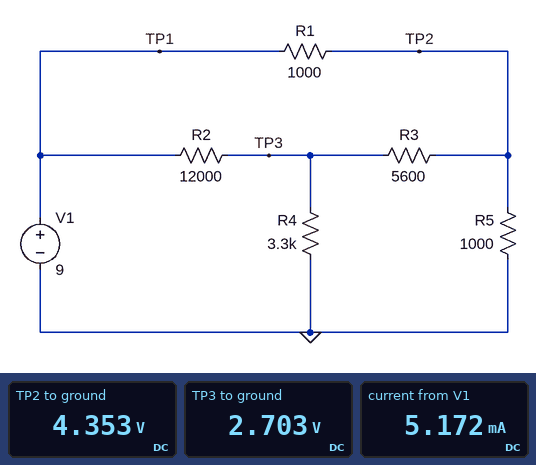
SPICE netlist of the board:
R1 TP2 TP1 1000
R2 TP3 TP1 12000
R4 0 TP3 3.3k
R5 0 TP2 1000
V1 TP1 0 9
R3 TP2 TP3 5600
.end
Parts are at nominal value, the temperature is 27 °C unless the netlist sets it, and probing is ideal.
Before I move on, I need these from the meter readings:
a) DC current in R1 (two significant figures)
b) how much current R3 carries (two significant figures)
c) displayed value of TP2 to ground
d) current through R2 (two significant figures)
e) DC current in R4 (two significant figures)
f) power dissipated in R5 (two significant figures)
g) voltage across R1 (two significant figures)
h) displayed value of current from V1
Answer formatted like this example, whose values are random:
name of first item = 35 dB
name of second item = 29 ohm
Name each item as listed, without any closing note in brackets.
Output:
DC current in R1 = 4.6 mA
how much current R3 carries = 290 µA
displayed value of TP2 to ground = 4.353 V
current through R2 = 520 µA
DC current in R4 = 820 µA
power dissipated in R5 = 19 mW
voltage across R1 = 4.6 V
displayed value of current from V1 = 5.172 mA
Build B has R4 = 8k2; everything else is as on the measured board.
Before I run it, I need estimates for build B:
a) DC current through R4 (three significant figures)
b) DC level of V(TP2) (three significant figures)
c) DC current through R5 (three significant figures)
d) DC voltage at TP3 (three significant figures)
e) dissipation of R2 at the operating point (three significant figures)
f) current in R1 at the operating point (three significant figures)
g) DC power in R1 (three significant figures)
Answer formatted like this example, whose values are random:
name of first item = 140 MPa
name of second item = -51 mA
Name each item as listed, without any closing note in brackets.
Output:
DC current through R4 = 491 µA
DC level of V(TP2) = 4.46 V
DC current through R5 = 4.46 mA
DC voltage at TP3 = 4.03 V
dissipation of R2 at the operating point = 2.06 mW
current in R1 at the operating point = 4.54 mA
DC power in R1 = 20.6 mW
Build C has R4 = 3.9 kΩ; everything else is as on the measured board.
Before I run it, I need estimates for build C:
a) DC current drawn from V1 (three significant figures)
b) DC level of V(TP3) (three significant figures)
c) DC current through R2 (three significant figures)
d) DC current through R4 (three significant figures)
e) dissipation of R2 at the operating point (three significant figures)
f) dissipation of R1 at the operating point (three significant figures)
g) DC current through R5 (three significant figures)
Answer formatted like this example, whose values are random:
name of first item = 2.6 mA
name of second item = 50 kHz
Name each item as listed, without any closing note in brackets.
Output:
DC current drawn from V1 = 5.13 mA
DC level of V(TP3) = 2.95 V
DC current through R2 = 504 µA
DC current through R4 = 757 µA
dissipation of R2 at the operating point = 3.05 mW
dissipation of R1 at the operating point = 21.4 mW
DC current through R5 = 4.37 mA
